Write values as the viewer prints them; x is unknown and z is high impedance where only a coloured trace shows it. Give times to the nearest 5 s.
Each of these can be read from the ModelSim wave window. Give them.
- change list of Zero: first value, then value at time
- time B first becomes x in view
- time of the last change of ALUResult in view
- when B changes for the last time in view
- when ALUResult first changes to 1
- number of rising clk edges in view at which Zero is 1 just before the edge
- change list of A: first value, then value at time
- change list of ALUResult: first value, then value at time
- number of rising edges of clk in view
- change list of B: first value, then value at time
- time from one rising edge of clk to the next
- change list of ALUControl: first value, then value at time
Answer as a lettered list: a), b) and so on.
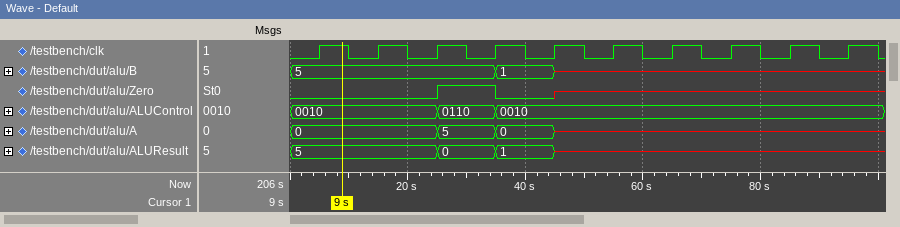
a) 0, 1 at 25 s, 0 at 35 s, x at 45 s
b) 45 s
c) 45 s
d) 45 s
e) 35 s
f) 1
g) 0, 5 at 25 s, 0 at 35 s, x at 45 s
h) 5, 0 at 25 s, 1 at 35 s, x at 45 s
i) 10
j) 5, 1 at 35 s, x at 45 s
k) 10 s
l) 0010, 0110 at 25 s, 0010 at 35 s
